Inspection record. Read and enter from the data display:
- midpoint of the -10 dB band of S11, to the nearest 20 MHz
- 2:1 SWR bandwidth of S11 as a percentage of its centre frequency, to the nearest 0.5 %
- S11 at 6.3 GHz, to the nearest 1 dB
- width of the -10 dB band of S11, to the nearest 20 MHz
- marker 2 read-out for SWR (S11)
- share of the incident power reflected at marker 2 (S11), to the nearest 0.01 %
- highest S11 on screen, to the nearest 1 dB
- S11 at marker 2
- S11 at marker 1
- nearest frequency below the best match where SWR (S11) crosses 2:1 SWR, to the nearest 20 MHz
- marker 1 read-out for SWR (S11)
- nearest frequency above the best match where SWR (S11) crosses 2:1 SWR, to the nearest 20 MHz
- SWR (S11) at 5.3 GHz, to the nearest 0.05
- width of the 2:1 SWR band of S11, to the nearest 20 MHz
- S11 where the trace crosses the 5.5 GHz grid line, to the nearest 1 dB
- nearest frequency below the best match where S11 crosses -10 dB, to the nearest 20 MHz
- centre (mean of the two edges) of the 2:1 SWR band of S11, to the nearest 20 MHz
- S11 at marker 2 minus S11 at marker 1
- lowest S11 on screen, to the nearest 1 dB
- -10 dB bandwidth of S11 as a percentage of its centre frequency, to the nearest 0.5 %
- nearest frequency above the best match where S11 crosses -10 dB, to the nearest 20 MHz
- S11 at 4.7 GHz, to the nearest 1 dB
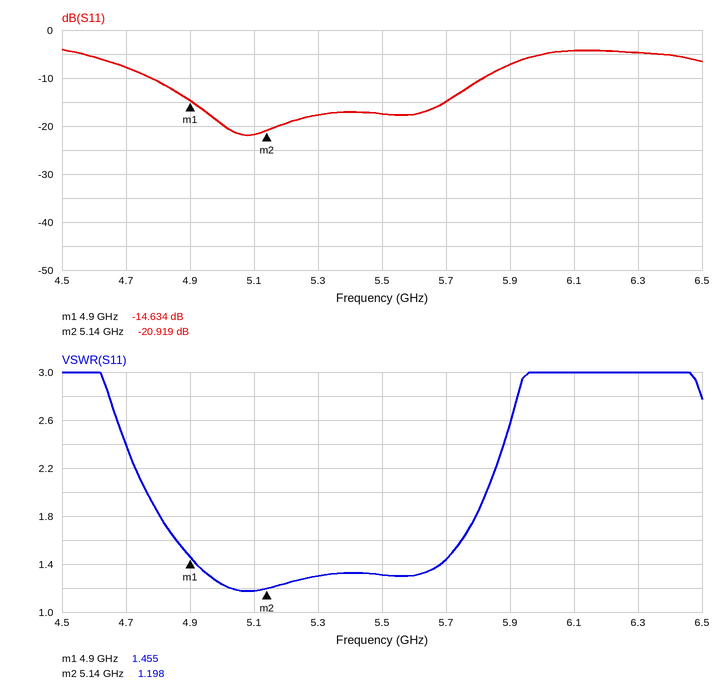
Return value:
5.30 GHz
20.0 %
-5 dB
1.04 GHz
1.198
0.81 %
-4 dB
-20.919 dB
-14.634 dB
4.76 GHz
1.455
5.82 GHz
1.30
1.06 GHz
-17 dB
4.78 GHz
5.30 GHz
-6.285 dB
-22 dB
19.5 %
5.82 GHz
-8 dB
